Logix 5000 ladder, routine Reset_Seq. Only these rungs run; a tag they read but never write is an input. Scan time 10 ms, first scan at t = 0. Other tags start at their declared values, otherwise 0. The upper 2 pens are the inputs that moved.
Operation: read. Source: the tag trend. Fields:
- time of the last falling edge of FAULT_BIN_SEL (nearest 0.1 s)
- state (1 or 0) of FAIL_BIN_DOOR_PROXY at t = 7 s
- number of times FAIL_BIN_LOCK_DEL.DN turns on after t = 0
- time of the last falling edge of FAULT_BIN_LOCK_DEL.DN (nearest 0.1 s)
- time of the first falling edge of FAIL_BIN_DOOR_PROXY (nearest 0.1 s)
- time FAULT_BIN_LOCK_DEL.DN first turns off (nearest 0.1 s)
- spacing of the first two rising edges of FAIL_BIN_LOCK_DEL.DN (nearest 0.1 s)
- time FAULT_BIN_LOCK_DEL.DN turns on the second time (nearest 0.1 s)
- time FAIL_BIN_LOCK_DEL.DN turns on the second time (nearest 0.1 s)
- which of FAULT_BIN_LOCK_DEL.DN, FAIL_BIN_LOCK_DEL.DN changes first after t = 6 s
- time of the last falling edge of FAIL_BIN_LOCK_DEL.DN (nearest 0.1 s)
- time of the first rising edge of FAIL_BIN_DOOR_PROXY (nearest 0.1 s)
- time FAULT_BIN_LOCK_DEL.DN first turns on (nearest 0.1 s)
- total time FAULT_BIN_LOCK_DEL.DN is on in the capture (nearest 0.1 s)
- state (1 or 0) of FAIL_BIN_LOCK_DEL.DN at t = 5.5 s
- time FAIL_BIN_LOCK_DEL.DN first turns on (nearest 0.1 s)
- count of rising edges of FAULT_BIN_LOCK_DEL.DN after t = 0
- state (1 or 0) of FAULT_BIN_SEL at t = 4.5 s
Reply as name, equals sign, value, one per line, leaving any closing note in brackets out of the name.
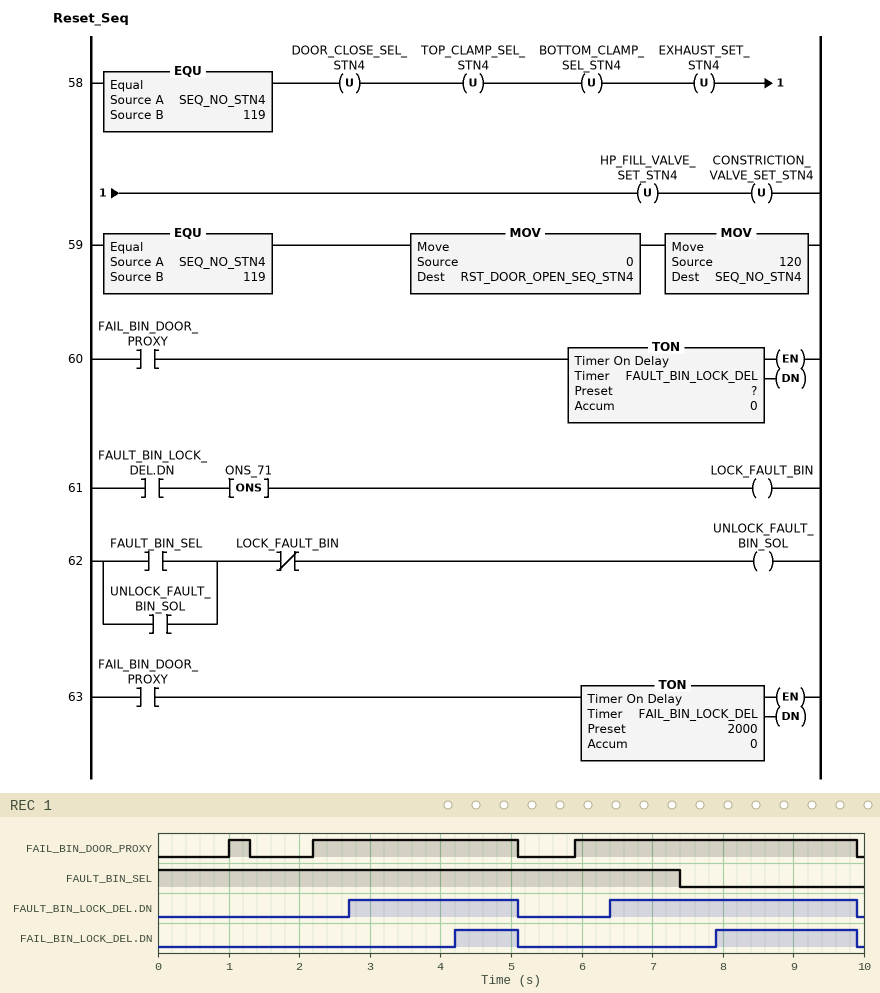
time of the last falling edge of FAULT_BIN_SEL = 7.4 s
state (1 or 0) of FAIL_BIN_DOOR_PROXY at t = 7 s = 1
number of times FAIL_BIN_LOCK_DEL.DN turns on after t = 0 = 2
time of the last falling edge of FAULT_BIN_LOCK_DEL.DN = 9.9 s
time of the first falling edge of FAIL_BIN_DOOR_PROXY = 1.3 s
time FAULT_BIN_LOCK_DEL.DN first turns off = 5.1 s
spacing of the first two rising edges of FAIL_BIN_LOCK_DEL.DN = 3.7 s
time FAULT_BIN_LOCK_DEL.DN turns on the second time = 6.4 s
time FAIL_BIN_LOCK_DEL.DN turns on the second time = 7.9 s
which of FAULT_BIN_LOCK_DEL.DN, FAIL_BIN_LOCK_DEL.DN changes first after t = 6 s = FAULT_BIN_LOCK_DEL.DN
time of the last falling edge of FAIL_BIN_LOCK_DEL.DN = 9.9 s
time of the first rising edge of FAIL_BIN_DOOR_PROXY = 1.0 s
time FAULT_BIN_LOCK_DEL.DN first turns on = 2.7 s
total time FAULT_BIN_LOCK_DEL.DN is on in the capture = 5.9 s
state (1 or 0) of FAIL_BIN_LOCK_DEL.DN at t = 5.5 s = 0
time FAIL_BIN_LOCK_DEL.DN first turns on = 4.2 s
count of rising edges of FAULT_BIN_LOCK_DEL.DN after t = 0 = 2
state (1 or 0) of FAULT_BIN_SEL at t = 4.5 s = 1
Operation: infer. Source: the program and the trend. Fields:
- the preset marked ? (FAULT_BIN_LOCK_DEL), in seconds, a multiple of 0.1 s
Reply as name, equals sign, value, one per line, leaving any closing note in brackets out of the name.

the preset marked ? (FAULT_BIN_LOCK_DEL), in seconds, a multiple of 0.1 s = 0.5 s
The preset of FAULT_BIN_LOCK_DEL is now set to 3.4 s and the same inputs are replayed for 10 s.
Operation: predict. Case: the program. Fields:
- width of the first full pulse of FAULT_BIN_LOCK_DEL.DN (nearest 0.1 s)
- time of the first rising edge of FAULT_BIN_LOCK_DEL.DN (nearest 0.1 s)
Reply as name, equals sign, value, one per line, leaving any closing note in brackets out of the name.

width of the first full pulse of FAULT_BIN_LOCK_DEL.DN = 0.6 s
time of the first rising edge of FAULT_BIN_LOCK_DEL.DN = 9.3 s
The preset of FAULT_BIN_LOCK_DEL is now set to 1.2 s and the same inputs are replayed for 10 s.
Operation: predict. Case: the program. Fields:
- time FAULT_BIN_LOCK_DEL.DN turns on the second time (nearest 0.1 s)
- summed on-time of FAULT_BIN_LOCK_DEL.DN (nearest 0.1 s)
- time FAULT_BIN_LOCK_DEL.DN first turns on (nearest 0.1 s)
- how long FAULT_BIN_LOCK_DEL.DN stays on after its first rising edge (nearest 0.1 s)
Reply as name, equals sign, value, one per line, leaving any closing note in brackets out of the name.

time FAULT_BIN_LOCK_DEL.DN turns on the second time = 7.1 s
summed on-time of FAULT_BIN_LOCK_DEL.DN = 4.5 s
time FAULT_BIN_LOCK_DEL.DN first turns on = 3.4 s
how long FAULT_BIN_LOCK_DEL.DN stays on after its first rising edge = 1.7 s
